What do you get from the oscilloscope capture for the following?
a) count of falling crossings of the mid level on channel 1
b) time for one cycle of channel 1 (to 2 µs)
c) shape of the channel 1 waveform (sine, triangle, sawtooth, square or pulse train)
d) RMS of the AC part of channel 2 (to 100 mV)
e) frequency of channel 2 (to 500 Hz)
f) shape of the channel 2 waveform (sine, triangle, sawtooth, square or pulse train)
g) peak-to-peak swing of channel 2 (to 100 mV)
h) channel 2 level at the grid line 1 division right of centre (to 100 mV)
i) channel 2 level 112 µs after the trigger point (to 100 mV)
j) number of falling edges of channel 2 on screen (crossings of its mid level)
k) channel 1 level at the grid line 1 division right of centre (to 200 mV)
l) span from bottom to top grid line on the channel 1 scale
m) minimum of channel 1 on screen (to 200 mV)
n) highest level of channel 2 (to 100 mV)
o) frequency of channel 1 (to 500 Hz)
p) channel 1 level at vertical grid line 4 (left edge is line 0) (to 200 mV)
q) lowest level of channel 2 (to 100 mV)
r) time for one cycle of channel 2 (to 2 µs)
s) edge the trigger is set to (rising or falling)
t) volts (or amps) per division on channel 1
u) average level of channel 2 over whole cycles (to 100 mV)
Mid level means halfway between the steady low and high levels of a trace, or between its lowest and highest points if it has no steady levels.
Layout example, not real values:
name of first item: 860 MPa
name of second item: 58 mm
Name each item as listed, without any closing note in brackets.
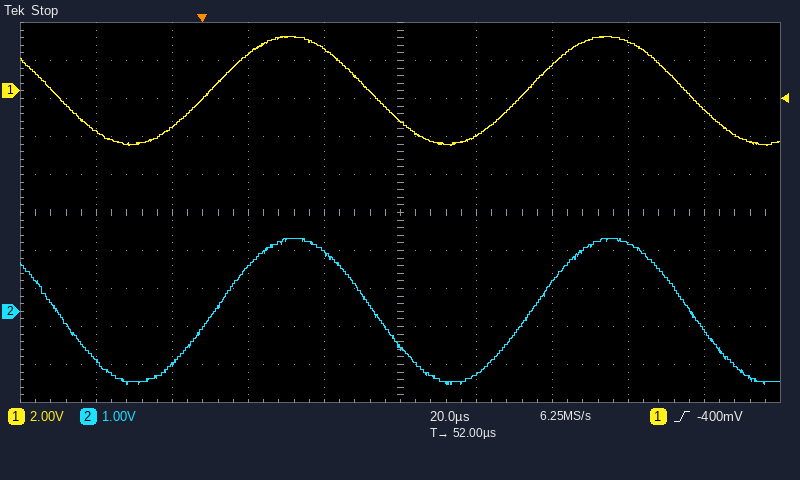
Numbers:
count of falling crossings of the mid level on channel 1: 3
time for one cycle of channel 1: 84 µs
shape of the channel 1 waveform: sine
RMS of the AC part of channel 2: 1.3 V
frequency of channel 2: 12.0 kHz
shape of the channel 2 waveform: sine
peak-to-peak swing of channel 2: 3.8 V
channel 2 level at the grid line 1 division right of centre: -1.7 V
channel 2 level 112 µs after the trigger point: 1.8 V
number of falling edges of channel 2 on screen: 3
channel 1 level at the grid line 1 division right of centre: -2.4 V
span from bottom to top grid line on the channel 1 scale: 20 V
minimum of channel 1 on screen: -2.8 V
highest level of channel 2: 1.9 V
frequency of channel 1: 12.0 kHz
channel 1 level at vertical grid line 4 (left edge is line 0): 2.2 V
lowest level of channel 2: -1.9 V
time for one cycle of channel 2: 84 µs
edge the trigger is set to: rising
volts (or amps) per division on channel 1: 2 V
average level of channel 2 over whole cycles: 0.0 V
